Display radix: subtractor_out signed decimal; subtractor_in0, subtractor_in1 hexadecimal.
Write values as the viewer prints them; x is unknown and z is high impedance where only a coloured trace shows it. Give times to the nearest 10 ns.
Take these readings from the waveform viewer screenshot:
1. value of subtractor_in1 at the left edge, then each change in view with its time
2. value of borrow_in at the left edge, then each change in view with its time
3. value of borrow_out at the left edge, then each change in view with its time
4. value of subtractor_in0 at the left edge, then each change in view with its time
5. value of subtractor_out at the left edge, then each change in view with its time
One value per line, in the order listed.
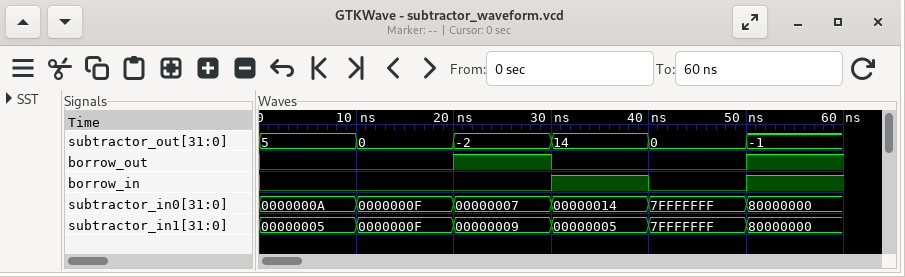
00000005, 0000000F at 10 ns, 00000009 at 20 ns, 00000005 at 30 ns, 7FFFFFFF at 40 ns, 80000000 at 50 ns
0, 1 at 30 ns, 0 at 40 ns, 1 at 50 ns
0, 1 at 20 ns, 0 at 30 ns, 1 at 50 ns
0000000A, 0000000F at 10 ns, 00000007 at 20 ns, 00000014 at 30 ns, 7FFFFFFF at 40 ns, 80000000 at 50 ns
5, 0 at 10 ns, -2 at 20 ns, 14 at 30 ns, 0 at 40 ns, -1 at 50 ns
